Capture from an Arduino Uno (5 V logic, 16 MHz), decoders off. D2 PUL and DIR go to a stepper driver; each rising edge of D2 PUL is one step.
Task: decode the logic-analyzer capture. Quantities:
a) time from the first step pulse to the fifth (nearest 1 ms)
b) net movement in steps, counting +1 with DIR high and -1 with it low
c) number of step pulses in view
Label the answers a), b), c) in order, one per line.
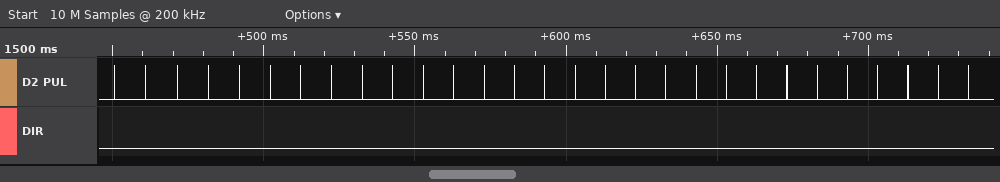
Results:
a) 41 ms
b) -29
c) 29
